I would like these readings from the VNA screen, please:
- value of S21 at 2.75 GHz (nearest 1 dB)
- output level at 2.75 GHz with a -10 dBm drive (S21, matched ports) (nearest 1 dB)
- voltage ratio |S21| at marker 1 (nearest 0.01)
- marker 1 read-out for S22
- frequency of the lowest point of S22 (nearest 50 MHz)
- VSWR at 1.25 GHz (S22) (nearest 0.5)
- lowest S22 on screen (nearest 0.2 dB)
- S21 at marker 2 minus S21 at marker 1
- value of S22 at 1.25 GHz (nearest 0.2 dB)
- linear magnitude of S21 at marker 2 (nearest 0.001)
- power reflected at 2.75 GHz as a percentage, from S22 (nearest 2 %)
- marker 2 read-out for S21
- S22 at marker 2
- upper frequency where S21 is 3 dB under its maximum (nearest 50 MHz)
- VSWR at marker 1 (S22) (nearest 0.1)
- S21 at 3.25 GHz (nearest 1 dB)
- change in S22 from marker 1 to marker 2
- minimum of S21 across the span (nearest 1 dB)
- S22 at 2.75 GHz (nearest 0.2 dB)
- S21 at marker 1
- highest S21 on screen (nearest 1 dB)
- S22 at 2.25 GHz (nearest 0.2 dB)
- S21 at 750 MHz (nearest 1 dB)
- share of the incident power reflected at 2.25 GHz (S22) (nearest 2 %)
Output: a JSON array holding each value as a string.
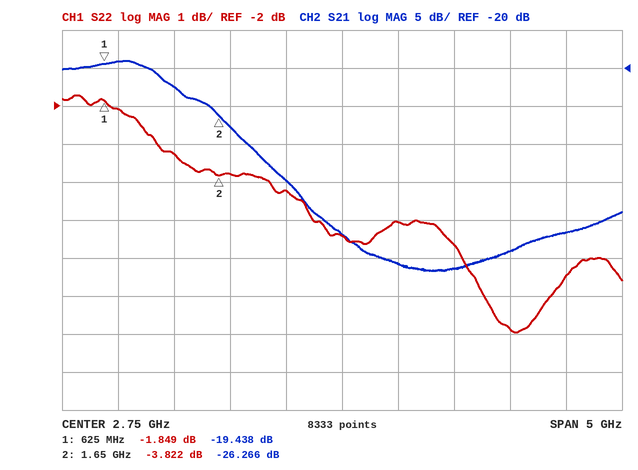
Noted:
["-42 dB", "-52 dBm", "0.11", "-1.849 dB", "4.30 GHz", "5.5", "-8.0 dB", "-6.828 dB", "-3.2 dB", "0.049", "28 %", "-26.266 dB", "-3.822 dB", "1.20 GHz", "9.4", "-46 dB", "-1.973 dB", "-47 dB", "-5.4 dB", "-19.438 dB", "-19 dB", "-4.2 dB", "-19 dB", "38 %"]
